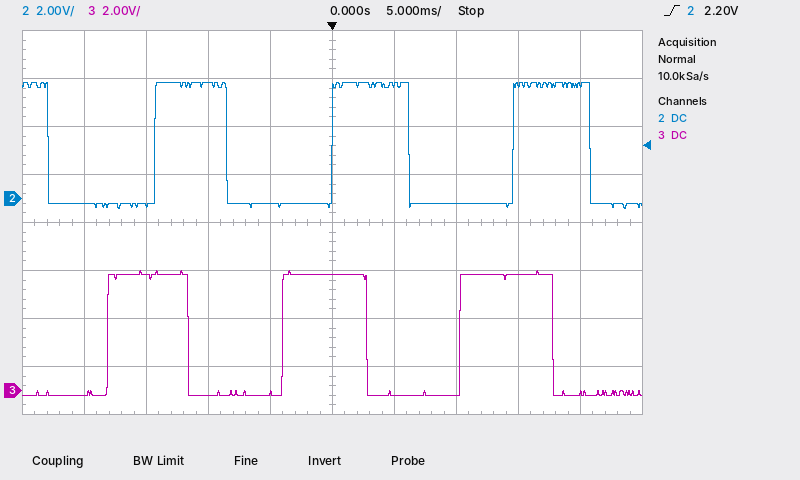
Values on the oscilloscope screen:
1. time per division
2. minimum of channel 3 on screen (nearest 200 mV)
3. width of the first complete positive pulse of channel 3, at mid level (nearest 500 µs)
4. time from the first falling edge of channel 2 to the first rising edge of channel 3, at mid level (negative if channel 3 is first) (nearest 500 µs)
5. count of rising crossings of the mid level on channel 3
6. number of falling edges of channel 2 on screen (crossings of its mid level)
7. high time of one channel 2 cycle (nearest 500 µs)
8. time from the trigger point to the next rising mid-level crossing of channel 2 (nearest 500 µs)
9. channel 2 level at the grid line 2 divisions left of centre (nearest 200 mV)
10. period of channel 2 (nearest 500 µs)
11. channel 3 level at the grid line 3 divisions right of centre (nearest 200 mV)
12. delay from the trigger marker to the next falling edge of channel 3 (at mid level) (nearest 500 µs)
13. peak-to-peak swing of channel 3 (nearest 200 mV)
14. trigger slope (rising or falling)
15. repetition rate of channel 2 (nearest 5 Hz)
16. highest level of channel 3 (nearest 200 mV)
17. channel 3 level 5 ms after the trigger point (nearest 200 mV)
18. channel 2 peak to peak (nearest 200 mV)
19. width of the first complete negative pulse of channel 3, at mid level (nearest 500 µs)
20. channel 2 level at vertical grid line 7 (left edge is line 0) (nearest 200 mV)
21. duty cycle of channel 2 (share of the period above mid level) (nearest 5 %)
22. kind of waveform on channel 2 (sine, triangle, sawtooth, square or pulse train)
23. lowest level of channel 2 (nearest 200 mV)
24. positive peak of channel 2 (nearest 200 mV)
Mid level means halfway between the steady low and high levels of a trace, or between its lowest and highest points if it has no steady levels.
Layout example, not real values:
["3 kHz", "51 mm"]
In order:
["5 ms", "-200 mV", "6.5 ms", "+5.0 ms", "3", "4", "6.0 ms", "14.5 ms", "4.8 V", "14.5 ms", "4.8 V", "3.0 ms", "5.2 V", "rising", "70 Hz", "5.0 V", "-200 mV", "5.2 V", "7.5 ms", "-200 mV", "40 %", "pulse train", "-400 mV", "4.8 V"]
